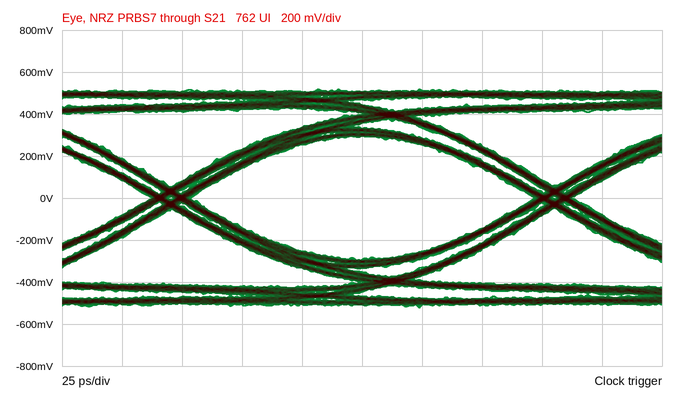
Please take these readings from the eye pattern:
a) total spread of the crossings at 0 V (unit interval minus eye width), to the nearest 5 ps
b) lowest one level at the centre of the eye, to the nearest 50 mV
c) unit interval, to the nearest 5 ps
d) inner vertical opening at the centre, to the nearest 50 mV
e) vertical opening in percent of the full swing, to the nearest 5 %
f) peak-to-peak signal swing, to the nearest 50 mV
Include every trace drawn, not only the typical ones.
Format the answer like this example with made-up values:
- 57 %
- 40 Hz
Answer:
- 15 ps
- 300 mV
- 160 ps
- 600 mV
- 55 %
- 1.05 V
